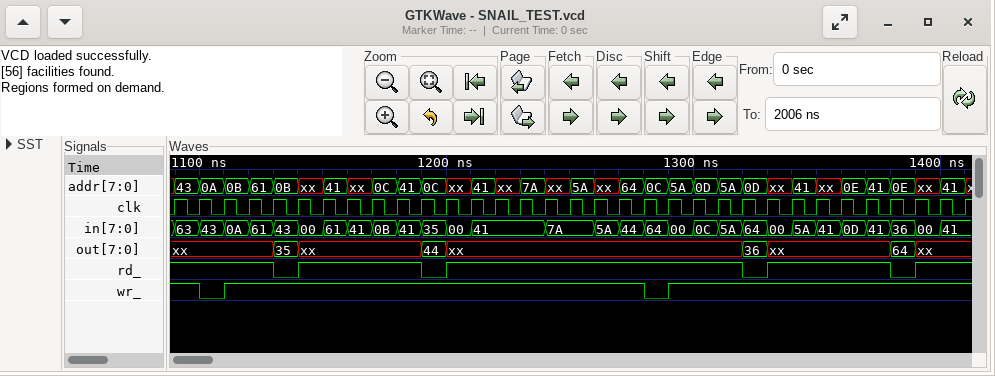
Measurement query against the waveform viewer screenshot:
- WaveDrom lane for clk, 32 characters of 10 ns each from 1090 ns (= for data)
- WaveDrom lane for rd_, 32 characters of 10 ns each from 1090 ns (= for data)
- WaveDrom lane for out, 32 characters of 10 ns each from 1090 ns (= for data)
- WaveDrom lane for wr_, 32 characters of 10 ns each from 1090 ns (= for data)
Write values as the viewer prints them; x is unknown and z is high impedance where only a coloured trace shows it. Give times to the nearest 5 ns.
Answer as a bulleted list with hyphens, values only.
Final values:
- {name: 'clk', wave: 'p...............................'}
- {name: 'rd_', wave: '1...01....01...........01....01.'}
- {name: 'out', wave: 'x...=x....=x...........=x....=x.', data: '35 44 36 64'}
- {name: 'wr_', wave: '101................01...........'}
